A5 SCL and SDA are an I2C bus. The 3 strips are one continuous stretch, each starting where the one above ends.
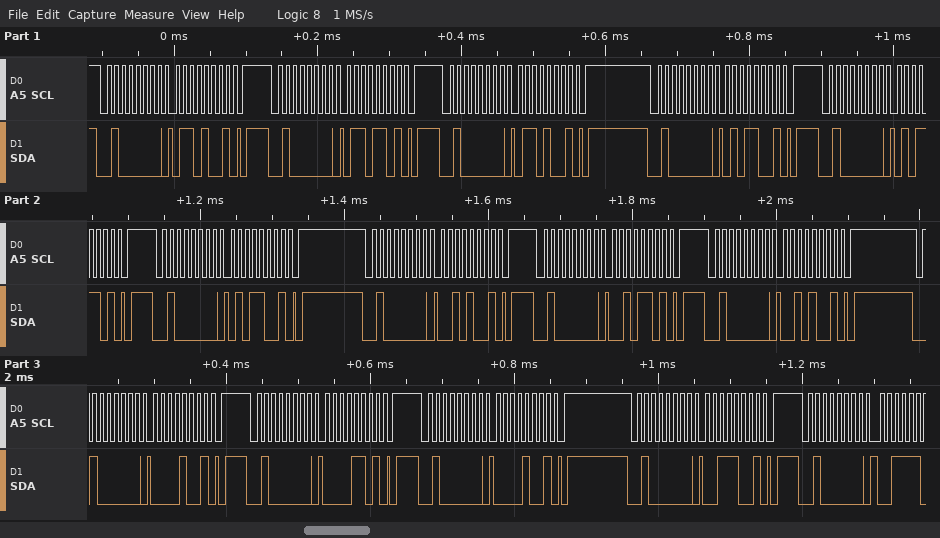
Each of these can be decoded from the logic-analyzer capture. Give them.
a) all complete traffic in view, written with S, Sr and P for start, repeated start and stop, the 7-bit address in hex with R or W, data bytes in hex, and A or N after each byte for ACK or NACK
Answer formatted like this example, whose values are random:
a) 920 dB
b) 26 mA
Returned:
a) S 20W A 69 A P S 20W A 6D A P S 20W A 69 A P S 20W A 59 A P S 20W A 5D A P S 20W A 59 A P S 20W A 29 A P S 20W A 2D A P S 20W A 29 A P S 20W A 09 A P S 20W A 0D A P S 20W A 09 A P S 20W A 39 A P S 20W A
